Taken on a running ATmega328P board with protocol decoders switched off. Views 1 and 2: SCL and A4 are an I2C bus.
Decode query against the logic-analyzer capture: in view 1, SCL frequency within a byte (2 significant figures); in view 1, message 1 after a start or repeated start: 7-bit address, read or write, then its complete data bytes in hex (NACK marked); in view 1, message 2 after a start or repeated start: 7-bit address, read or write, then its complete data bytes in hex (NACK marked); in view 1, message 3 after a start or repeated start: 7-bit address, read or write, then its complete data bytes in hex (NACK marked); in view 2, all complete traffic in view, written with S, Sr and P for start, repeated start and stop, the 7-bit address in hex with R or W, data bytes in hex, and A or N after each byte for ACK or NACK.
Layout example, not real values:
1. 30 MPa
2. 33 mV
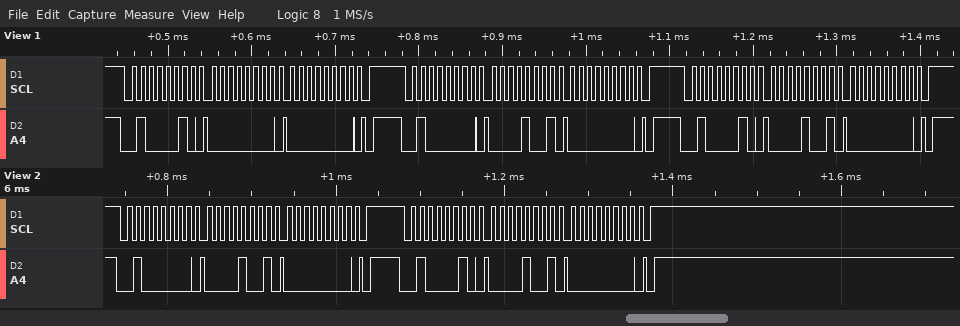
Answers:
1. 100 kHz
2. 0x21 write: 00 00
3. 0x20 write: 09 00
4. 0x21 write: 09 00
5. S 20W A 09 A 00 A P S 21W A 09 A 00 A P
